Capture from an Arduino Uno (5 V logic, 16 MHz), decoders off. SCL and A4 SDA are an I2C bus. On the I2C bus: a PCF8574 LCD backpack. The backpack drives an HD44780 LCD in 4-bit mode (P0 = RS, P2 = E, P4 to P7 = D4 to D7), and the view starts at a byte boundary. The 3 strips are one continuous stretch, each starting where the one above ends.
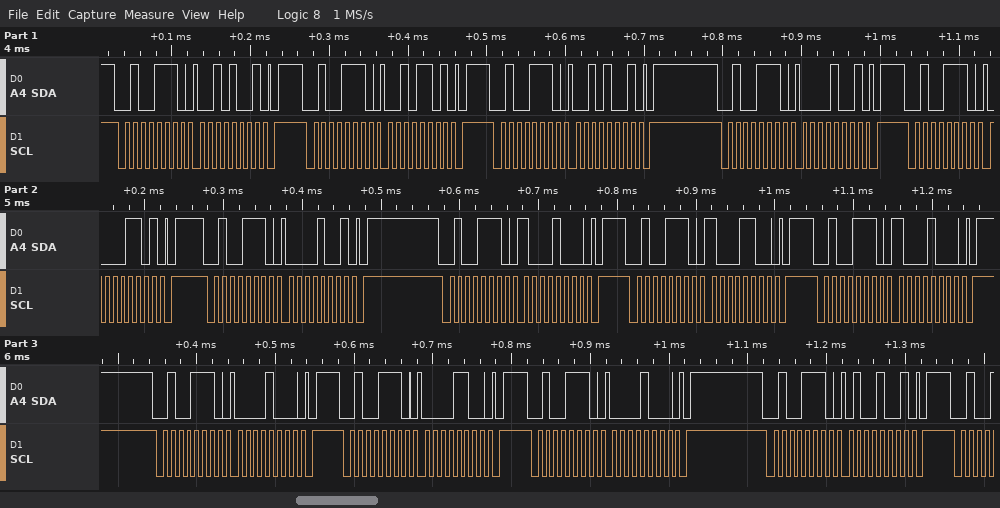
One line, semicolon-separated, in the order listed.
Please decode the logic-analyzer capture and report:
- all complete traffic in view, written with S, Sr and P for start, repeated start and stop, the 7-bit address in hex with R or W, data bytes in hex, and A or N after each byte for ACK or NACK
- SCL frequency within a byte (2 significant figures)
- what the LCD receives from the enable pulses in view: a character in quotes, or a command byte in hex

S 27W A 29 A P S 27W A 2D A P S 27W A 29 A P S 27W A 09 A P S 27W A 0D A P S 27W A 09 A P S 27W A 88 A P S 27W A 8C A P S 27W A 88 A P S 27W A 08 A P S 27W A 0C A P S 27W A 08 A P S 27W A 49 A P; 100 kHz; ' ' 0x80
